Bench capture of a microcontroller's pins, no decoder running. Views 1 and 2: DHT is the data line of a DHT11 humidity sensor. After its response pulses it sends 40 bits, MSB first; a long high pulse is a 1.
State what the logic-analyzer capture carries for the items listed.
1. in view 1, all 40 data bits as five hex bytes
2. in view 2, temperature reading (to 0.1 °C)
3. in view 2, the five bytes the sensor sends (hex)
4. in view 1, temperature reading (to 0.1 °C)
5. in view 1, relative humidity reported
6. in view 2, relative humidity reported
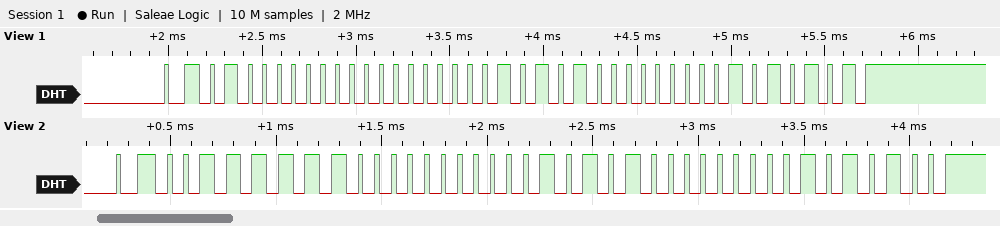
40 00 15 00 55
21.0 °C
3F 00 15 00 54
21.0 °C
64 %
63 %
